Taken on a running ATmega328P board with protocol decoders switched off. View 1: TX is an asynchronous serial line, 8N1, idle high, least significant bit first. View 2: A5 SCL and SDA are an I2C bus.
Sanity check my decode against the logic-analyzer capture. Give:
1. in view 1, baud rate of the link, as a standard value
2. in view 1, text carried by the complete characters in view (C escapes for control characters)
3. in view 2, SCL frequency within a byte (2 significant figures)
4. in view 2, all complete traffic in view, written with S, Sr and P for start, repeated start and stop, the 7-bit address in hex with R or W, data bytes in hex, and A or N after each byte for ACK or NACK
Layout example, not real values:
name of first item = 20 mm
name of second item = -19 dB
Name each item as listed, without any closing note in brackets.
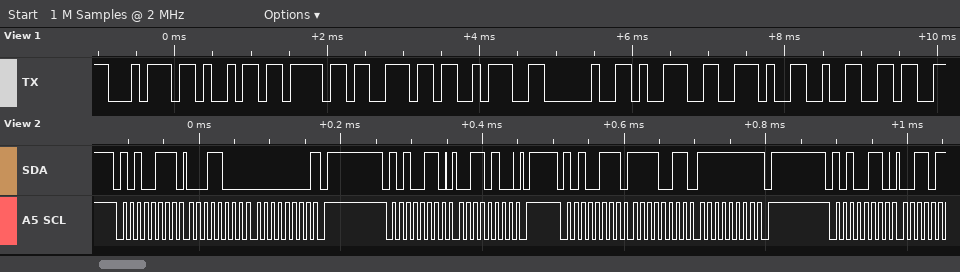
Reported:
in view 1, baud rate of the link, as a standard value = 9600 baud
in view 1, text carried by the complete characters in view = "tion: 9.2"
in view 2, SCL frequency within a byte = 100 kHz
in view 2, all complete traffic in view, written with S, Sr and P for start, repeated start and stop, the 7-bit address in hex with R or W, data bytes in hex, and A or N after each byte for ACK or NACK = S 53R A 18 A 00 N P S 53W A 34 A P S 53R A F3 A FF N P S 53W A
